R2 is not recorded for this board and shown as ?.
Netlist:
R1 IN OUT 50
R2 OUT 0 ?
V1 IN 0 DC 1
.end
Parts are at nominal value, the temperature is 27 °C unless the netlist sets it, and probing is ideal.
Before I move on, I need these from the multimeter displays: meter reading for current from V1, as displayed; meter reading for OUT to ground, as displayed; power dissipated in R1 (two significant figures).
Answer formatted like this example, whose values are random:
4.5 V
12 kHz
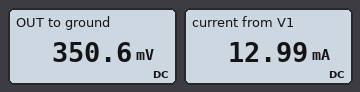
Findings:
12.99 mA
350.6 mV
8.4 mW
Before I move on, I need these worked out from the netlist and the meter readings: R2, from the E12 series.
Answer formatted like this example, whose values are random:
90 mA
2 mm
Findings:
27 Ω
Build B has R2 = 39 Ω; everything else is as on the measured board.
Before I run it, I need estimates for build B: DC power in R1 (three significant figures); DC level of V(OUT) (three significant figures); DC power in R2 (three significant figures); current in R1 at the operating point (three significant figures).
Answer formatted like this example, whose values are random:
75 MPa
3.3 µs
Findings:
6.31 mW
438 mV
4.92 mW
11.2 mA
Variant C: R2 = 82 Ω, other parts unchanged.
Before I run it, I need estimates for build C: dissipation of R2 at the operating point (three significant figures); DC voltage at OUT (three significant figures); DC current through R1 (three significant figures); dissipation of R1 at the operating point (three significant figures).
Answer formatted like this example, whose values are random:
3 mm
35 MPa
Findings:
4.71 mW
621 mV
7.58 mA
2.87 mW
